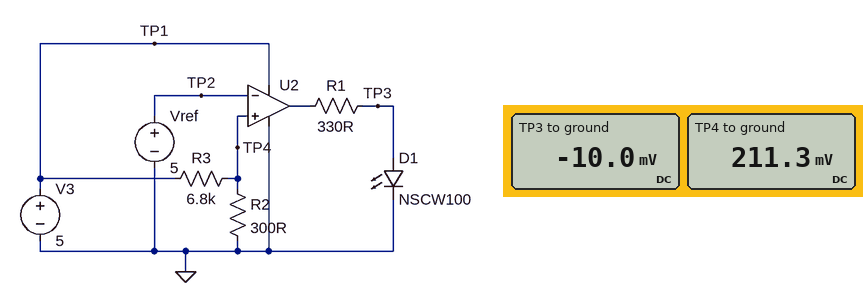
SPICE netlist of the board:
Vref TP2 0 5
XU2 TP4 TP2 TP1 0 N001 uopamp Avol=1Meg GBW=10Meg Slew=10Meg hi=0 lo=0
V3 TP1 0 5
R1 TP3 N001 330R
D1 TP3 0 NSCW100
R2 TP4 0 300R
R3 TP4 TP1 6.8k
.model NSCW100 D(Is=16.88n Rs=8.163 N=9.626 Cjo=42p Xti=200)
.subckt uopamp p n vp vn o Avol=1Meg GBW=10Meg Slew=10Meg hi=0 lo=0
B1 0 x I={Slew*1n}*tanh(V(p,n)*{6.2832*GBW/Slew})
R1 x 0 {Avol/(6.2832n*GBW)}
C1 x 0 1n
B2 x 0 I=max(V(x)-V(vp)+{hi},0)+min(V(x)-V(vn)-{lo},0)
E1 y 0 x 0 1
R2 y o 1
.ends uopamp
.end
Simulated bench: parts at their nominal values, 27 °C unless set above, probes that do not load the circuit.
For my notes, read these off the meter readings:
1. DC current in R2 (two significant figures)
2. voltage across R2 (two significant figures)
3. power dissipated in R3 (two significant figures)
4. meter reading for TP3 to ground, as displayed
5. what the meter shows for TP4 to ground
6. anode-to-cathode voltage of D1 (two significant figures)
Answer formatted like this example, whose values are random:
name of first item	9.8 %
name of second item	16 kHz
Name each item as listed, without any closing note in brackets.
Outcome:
DC current in R2	700 µA
voltage across R2	210 mV
power dissipated in R3	3.4 mW
meter reading for TP3 to ground, as displayed	-10.0 mV
what the meter shows for TP4 to ground	211.3 mV
anode-to-cathode voltage of D1	-10 mV
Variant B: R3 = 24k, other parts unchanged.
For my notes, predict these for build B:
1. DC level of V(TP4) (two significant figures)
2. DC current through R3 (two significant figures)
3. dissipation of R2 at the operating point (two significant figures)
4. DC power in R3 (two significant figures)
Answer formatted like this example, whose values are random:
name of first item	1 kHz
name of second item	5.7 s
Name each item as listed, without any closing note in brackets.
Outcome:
DC level of V(TP4)	62 mV
DC current through R3	210 µA
dissipation of R2 at the operating point	13 µW
DC power in R3	1.0 mW
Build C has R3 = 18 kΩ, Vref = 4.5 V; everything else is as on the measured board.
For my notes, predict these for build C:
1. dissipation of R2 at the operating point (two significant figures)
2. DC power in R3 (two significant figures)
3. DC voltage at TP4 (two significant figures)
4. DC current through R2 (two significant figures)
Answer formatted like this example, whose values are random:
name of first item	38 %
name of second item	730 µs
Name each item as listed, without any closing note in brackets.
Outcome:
dissipation of R2 at the operating point	22 µW
DC power in R3	1.3 mW
DC voltage at TP4	82 mV
DC current through R2	270 µA
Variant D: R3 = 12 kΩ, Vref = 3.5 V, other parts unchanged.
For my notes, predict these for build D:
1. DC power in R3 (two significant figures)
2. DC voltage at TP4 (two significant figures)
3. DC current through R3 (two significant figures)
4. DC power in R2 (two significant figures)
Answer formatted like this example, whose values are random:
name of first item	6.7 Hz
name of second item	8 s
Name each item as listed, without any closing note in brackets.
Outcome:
DC power in R3	2.0 mW
DC voltage at TP4	120 mV
DC current through R3	410 µA
DC power in R2	50 µW
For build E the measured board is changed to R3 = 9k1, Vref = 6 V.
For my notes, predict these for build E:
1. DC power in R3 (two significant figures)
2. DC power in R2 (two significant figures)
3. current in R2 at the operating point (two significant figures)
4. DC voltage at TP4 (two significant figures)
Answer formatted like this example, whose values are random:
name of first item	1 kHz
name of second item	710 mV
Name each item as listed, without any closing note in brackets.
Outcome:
DC power in R3	2.6 mW
DC power in R2	85 µW
current in R2 at the operating point	530 µA
DC voltage at TP4	160 mV
